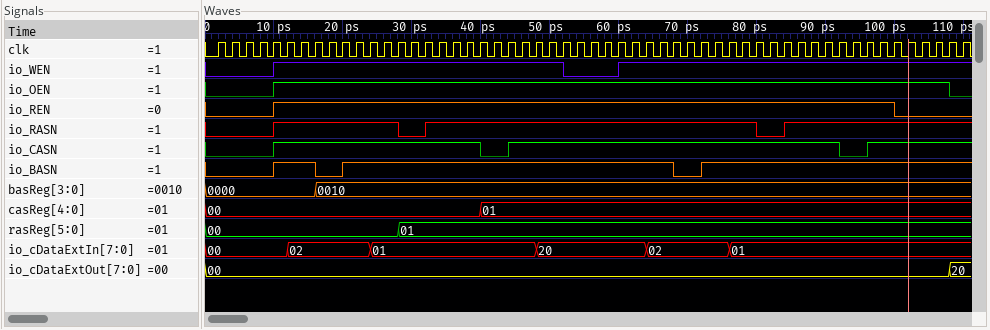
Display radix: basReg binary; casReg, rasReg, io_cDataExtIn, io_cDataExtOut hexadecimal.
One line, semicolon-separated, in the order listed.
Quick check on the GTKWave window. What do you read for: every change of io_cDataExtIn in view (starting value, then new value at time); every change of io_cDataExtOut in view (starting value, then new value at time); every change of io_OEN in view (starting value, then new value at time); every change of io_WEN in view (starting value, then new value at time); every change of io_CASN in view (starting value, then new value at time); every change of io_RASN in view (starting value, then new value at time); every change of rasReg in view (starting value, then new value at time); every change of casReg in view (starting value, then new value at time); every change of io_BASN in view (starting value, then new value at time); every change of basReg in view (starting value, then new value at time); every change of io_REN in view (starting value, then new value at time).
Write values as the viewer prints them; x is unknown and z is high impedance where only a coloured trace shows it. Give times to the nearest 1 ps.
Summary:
00, 02 at 12 ps, 01 at 24 ps, 20 at 48 ps, 02 at 64 ps, 01 at 76 ps; 00, 20 at 108 ps; 0, 1 at 10 ps, 0 at 108 ps; 0, 1 at 10 ps, 0 at 52 ps, 1 at 60 ps; 0, 1 at 10 ps, 0 at 40 ps, 1 at 44 ps, 0 at 92 ps, 1 at 96 ps; 0, 1 at 10 ps, 0 at 28 ps, 1 at 32 ps, 0 at 80 ps, 1 at 84 ps; 00, 01 at 28 ps; 00, 01 at 40 ps; 0, 1 at 10 ps, 0 at 16 ps, 1 at 20 ps, 0 at 68 ps, 1 at 72 ps; 0000, 0010 at 16 ps; 0, 1 at 10 ps, 0 at 100 ps
